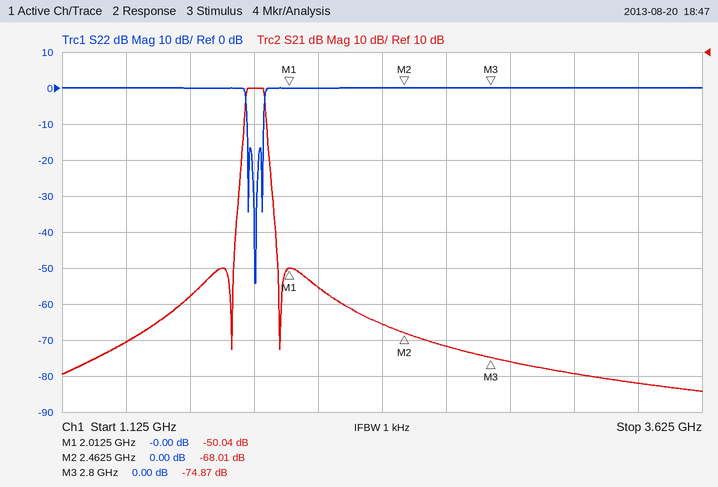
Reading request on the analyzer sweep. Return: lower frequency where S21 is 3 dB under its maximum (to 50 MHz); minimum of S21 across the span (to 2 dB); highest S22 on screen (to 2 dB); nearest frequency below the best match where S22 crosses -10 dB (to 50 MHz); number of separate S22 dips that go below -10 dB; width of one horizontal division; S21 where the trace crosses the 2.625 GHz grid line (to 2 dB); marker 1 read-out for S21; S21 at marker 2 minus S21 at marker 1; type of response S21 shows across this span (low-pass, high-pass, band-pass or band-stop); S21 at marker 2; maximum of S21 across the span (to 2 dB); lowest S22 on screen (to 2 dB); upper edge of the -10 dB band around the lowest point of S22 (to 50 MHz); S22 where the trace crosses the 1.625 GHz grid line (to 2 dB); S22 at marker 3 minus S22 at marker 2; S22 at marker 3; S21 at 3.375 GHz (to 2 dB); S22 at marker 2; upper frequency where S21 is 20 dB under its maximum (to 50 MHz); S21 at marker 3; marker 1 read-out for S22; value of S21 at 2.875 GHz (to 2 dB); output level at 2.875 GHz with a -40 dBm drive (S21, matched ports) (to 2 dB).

1.85 GHz
-84 dB
0 dB
1.85 GHz
3
250 MHz
-72 dB
-50.04 dB
-17.97 dB
band-pass
-68.01 dB
0 dB
-54 dB
1.90 GHz
0 dB
0.00 dB
0.00 dB
-82 dB
0.00 dB
1.95 GHz
-74.87 dB
-0.00 dB
-76 dB
-116 dBm
